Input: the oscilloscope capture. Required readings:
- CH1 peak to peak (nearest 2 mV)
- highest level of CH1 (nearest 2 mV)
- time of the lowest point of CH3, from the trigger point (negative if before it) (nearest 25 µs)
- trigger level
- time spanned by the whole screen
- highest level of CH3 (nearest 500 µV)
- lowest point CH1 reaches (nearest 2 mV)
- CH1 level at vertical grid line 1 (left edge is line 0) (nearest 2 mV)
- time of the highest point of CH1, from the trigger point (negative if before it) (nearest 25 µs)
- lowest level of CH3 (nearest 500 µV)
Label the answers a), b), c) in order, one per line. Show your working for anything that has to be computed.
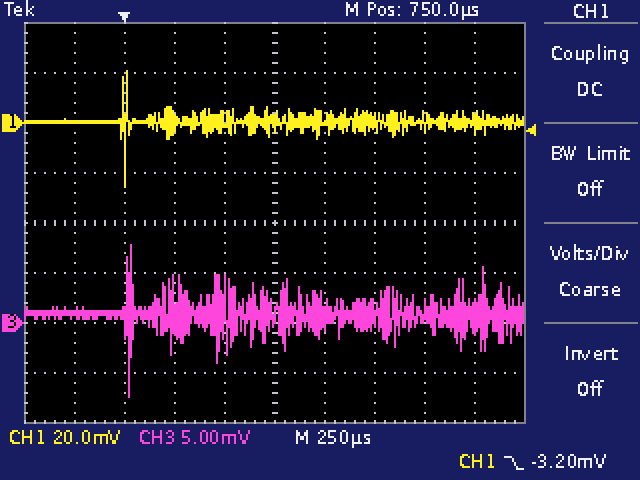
a) 20 mV − (-26 mV) = 46 mV
b) 20 mV
c) +25 µs
d) -3.20 mV
e) 2.5 ms
f) 8.0 mV
g) -26 mV
h) 0 mV
i) +25 µs
j) -7.5 mV
